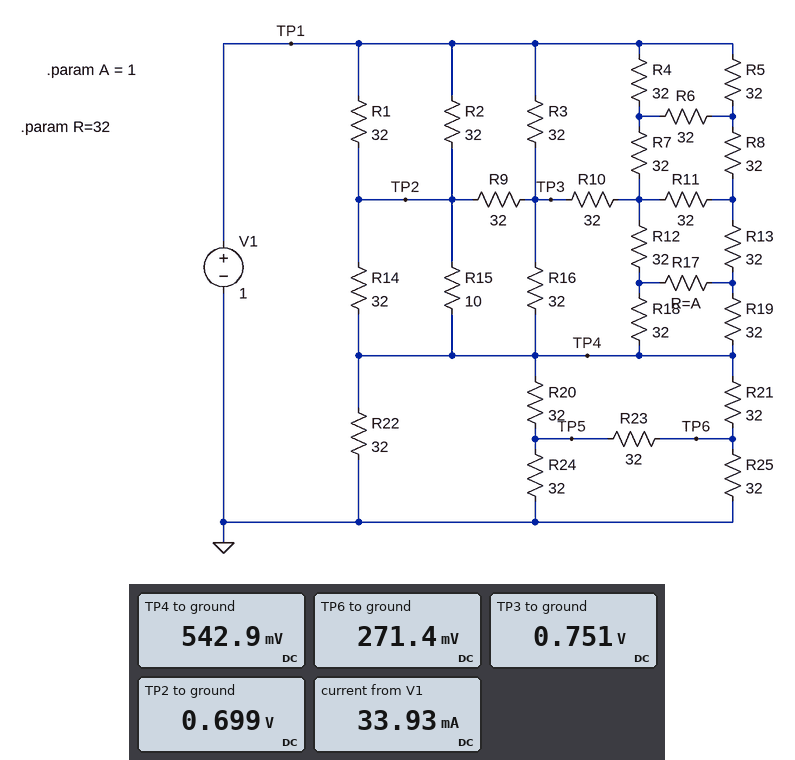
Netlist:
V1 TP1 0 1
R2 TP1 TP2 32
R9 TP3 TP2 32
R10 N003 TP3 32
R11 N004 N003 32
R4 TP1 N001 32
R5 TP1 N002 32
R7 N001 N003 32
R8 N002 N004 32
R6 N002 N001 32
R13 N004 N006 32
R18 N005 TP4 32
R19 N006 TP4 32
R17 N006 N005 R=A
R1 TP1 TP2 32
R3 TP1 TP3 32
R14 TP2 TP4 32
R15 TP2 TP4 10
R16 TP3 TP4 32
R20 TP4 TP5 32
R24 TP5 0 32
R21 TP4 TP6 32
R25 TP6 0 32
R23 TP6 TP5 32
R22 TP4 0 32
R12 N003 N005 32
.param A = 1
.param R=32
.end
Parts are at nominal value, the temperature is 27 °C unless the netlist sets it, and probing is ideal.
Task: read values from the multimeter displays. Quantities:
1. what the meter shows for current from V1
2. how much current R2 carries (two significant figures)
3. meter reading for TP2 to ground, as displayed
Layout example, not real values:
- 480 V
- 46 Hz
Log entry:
- 33.93 mA
- 9.4 mA
- 0.699 V
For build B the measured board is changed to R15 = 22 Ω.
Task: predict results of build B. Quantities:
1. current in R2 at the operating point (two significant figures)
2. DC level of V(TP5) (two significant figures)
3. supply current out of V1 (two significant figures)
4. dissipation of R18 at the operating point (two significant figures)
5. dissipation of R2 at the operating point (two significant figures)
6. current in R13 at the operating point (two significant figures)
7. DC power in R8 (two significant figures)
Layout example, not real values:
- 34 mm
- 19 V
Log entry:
- 8.3 mA
- 260 mV
- 32 mA
- 460 µW
- 2.2 mW
- 3.8 mA
- 470 µW
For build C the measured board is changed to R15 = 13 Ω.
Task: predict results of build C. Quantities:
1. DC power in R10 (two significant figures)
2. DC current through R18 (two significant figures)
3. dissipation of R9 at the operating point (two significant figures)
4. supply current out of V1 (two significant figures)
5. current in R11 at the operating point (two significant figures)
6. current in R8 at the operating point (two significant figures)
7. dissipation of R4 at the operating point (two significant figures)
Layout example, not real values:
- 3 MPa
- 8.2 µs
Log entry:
- 2.7 µW
- 3.6 mA
- 50 µW
- 33 mA
- 78 µA
- 3.7 mA
- 450 µW
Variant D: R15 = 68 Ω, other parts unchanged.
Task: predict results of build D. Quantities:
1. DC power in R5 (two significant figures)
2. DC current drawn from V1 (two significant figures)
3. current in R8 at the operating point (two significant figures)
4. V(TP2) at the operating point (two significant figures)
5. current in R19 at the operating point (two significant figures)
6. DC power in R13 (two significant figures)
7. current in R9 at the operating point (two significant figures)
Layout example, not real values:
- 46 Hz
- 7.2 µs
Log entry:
- 520 µW
- 30 mA
- 4.0 mA
- 770 mV
- 4.1 mA
- 530 µW
- 740 µA
